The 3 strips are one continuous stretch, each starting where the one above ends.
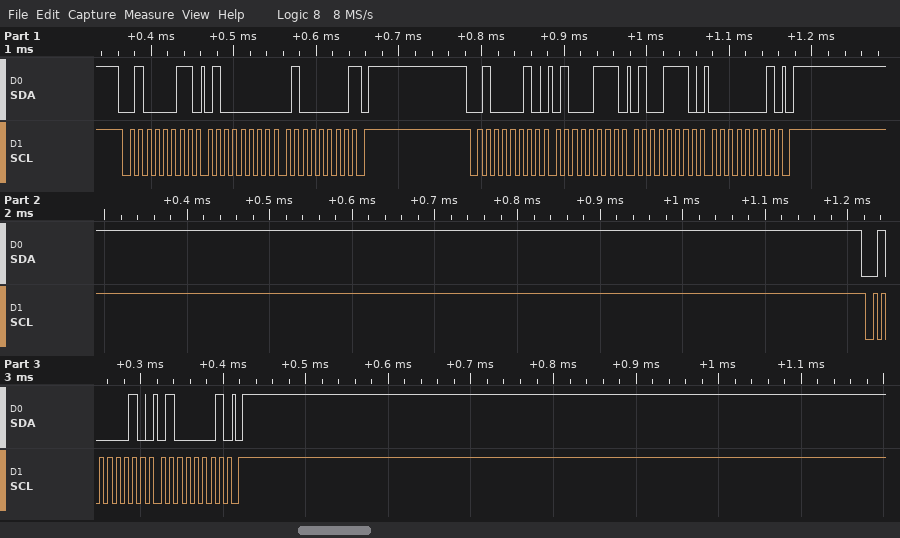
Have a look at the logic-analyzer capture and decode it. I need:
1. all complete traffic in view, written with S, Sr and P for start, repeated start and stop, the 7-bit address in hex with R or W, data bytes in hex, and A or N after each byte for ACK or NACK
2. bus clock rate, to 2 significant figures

S 21R A 40 A 40 N P S 21W A 47 A 4E A 01 A P S 21W A 41 A P
100 kHz
